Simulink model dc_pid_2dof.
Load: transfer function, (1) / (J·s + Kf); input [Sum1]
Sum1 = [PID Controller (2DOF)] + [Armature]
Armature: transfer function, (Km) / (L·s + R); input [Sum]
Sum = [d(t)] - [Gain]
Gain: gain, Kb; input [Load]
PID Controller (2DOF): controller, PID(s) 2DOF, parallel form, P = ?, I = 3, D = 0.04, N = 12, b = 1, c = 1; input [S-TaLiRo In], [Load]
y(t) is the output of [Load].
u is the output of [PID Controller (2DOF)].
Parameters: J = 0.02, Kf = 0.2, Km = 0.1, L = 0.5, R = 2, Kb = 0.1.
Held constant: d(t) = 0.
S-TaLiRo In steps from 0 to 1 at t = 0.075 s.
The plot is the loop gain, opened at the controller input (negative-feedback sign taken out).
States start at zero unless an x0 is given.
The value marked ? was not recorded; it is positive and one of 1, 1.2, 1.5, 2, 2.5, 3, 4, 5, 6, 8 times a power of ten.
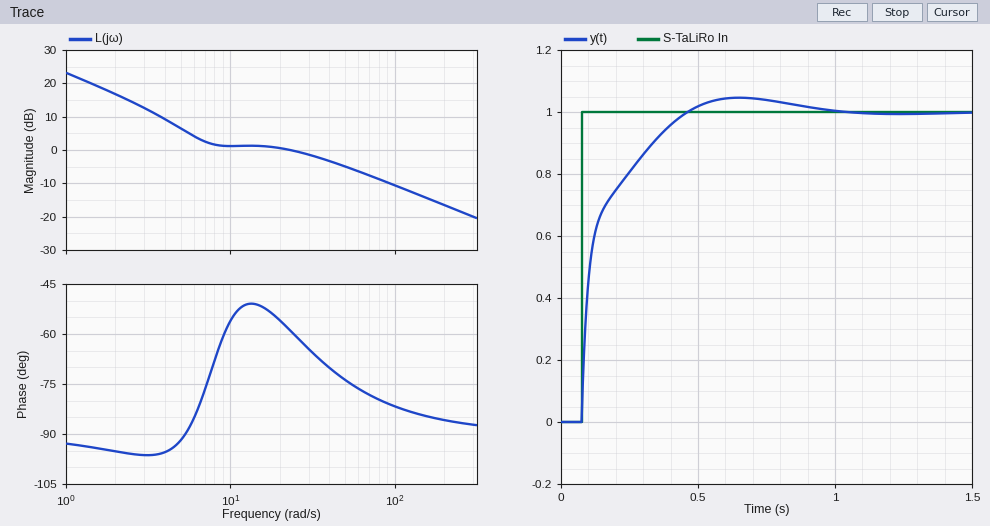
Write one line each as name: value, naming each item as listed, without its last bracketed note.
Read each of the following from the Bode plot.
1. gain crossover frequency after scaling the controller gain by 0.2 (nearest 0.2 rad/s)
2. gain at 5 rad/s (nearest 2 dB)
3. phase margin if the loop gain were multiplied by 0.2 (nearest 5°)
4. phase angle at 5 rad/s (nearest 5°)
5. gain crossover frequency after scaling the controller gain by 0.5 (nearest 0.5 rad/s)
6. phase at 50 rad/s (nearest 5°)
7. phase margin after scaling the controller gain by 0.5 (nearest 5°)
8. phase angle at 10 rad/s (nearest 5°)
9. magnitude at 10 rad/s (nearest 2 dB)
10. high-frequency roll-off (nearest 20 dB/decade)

gain crossover frequency after scaling the controller gain by 0.2: 2.6 rad/s
gain at 5 rad/s: 6 dB
phase margin if the loop gain were multiplied by 0.2: 85°
phase angle at 5 rad/s: -90°
gain crossover frequency after scaling the controller gain by 0.5: 5.0 rad/s
phase at 50 rad/s: -75°
phase margin after scaling the controller gain by 0.5: 90°
phase angle at 10 rad/s: -55°
magnitude at 10 rad/s: 2 dB
high-frequency roll-off: -20 dB/decade
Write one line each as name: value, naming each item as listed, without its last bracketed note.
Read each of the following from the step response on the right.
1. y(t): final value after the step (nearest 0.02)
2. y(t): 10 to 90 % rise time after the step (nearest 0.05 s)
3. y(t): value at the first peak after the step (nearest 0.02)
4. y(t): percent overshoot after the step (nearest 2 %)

y(t): final value after the step: 1.00
y(t): 10 to 90 % rise time after the step: 0.25 s
y(t): value at the first peak after the step: 1.04
y(t): percent overshoot after the step: 4 %
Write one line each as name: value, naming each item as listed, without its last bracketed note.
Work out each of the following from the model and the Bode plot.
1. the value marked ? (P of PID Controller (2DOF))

the value marked ? (P of PID Controller (2DOF)): 0.12
